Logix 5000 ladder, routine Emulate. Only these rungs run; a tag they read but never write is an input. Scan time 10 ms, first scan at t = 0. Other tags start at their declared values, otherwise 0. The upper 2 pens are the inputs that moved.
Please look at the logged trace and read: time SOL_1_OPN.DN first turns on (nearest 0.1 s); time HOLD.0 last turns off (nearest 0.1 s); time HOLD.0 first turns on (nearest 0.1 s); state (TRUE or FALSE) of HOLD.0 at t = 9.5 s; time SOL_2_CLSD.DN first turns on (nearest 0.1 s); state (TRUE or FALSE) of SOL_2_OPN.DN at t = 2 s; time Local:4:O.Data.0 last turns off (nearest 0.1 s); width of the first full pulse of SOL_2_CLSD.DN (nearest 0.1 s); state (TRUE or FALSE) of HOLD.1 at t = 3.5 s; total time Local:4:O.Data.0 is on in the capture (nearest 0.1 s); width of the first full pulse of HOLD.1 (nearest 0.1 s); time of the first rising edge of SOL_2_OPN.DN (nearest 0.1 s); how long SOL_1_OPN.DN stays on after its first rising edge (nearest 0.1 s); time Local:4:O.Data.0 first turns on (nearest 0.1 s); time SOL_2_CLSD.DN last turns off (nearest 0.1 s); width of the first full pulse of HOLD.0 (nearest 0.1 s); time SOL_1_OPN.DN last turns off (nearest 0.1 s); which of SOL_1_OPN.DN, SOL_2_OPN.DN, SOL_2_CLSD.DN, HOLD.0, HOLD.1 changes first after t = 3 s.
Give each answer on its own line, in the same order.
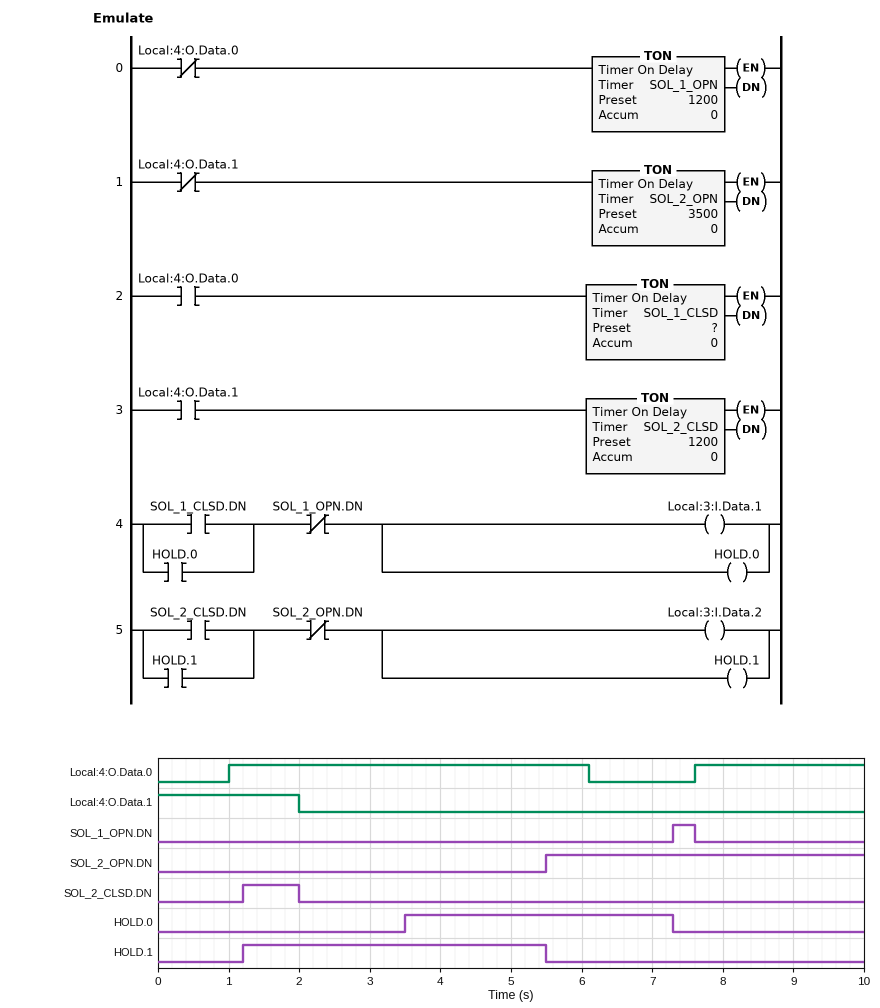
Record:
7.3 s
7.3 s
3.5 s
FALSE
1.2 s
FALSE
6.1 s
0.8 s
TRUE
7.5 s
4.3 s
5.5 s
0.3 s
1.0 s
2.0 s
3.8 s
7.6 s
HOLD.0
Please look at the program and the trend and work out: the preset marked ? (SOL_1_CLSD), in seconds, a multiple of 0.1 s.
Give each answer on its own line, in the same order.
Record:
2.5 s
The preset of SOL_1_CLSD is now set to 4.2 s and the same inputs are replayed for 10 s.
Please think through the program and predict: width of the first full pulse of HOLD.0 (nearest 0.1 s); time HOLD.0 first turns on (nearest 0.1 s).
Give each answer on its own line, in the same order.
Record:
2.1 s
5.2 s
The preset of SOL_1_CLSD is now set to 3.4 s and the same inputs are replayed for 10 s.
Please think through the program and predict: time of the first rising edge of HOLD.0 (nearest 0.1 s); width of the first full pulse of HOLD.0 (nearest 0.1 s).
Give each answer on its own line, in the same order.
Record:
4.4 s
2.9 s
